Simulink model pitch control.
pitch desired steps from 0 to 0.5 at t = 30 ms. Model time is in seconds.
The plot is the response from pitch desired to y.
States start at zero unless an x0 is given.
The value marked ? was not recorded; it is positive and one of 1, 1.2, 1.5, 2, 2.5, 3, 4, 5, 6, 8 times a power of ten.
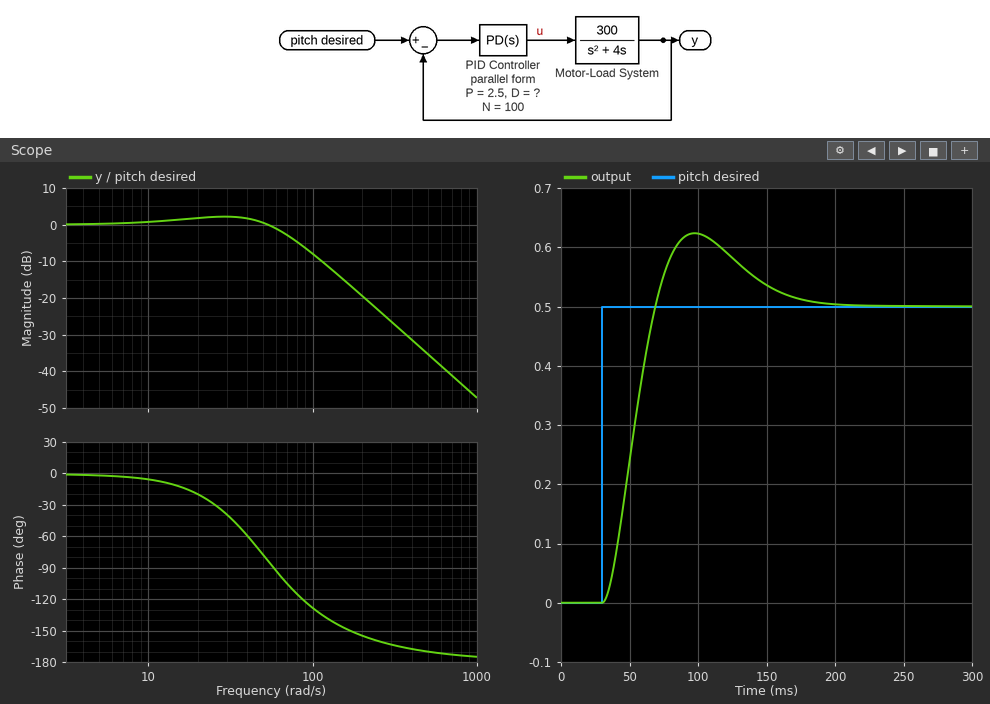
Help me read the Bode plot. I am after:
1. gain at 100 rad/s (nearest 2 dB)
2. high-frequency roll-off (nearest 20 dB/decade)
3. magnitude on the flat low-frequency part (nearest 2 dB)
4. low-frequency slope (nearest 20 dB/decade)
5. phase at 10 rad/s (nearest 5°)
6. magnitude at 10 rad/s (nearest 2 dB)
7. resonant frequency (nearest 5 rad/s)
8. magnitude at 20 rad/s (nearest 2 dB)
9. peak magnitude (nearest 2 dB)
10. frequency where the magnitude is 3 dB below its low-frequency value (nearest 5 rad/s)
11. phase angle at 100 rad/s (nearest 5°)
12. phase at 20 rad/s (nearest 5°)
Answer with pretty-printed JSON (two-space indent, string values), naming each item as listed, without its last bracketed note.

{
  "gain at 100 rad/s": "-8 dB",
  "high-frequency roll-off": "-40 dB/decade",
  "magnitude on the flat low-frequency part": "0 dB",
  "low-frequency slope": "0 dB/decade",
  "phase at 10 rad/s": "-5°",
  "magnitude at 10 rad/s": "0 dB",
  "resonant frequency": "30 rad/s",
  "magnitude at 20 rad/s": "2 dB",
  "peak magnitude": "2 dB",
  "frequency where the magnitude is 3 dB below its low-frequency value": "70 rad/s",
  "phase angle at 100 rad/s": "-130°",
  "phase at 20 rad/s": "-20°"
}
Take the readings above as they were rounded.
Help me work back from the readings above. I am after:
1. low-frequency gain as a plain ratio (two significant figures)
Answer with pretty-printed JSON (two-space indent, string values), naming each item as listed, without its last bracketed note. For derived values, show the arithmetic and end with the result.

{
  "low-frequency gain as a plain ratio": "10^(0 / 20) = 1.0"
}
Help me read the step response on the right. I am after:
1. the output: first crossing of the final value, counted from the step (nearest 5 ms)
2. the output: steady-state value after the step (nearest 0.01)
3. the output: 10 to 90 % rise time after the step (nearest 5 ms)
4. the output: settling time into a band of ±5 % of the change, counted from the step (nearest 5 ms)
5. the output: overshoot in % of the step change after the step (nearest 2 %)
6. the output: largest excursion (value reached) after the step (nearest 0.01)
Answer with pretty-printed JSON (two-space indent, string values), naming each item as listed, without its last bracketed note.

{
  "the output: first crossing of the final value, counted from the step": "40 ms",
  "the output: steady-state value after the step": "0.50",
  "the output: 10 to 90 % rise time after the step": "25 ms",
  "the output: settling time into a band of ±5 % of the change, counted from the step": "130 ms",
  "the output: overshoot in % of the step change after the step": "24 %",
  "the output: largest excursion (value reached) after the step": "0.62"
}
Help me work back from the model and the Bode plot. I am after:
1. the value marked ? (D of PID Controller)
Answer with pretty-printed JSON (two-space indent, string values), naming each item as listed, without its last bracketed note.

{
  "the value marked ?": "0.12"
}
